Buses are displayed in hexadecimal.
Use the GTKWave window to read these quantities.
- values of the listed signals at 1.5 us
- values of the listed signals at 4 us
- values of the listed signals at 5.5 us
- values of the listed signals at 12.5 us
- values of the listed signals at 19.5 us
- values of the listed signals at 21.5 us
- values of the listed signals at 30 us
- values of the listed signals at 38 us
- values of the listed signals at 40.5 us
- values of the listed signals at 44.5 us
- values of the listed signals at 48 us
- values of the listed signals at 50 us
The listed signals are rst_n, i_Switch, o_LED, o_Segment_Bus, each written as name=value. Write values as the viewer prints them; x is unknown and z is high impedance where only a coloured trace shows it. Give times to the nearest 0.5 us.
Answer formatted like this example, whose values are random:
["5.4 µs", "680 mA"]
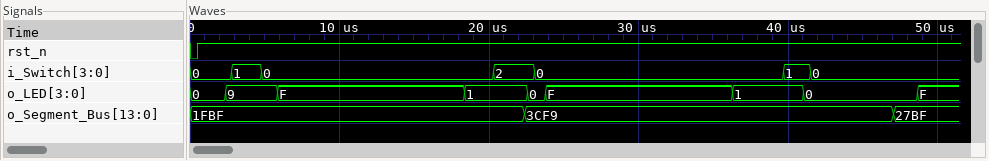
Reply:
["rst_n=1, i_Switch=0, o_LED=0, o_Segment_Bus=1FBF", "rst_n=1, i_Switch=1, o_LED=9, o_Segment_Bus=1FBF", "rst_n=1, i_Switch=0, o_LED=9, o_Segment_Bus=1FBF", "rst_n=1, i_Switch=0, o_LED=F, o_Segment_Bus=1FBF", "rst_n=1, i_Switch=0, o_LED=1, o_Segment_Bus=1FBF", "rst_n=1, i_Switch=2, o_LED=1, o_Segment_Bus=1FBF", "rst_n=1, i_Switch=0, o_LED=F, o_Segment_Bus=3CF9", "rst_n=1, i_Switch=0, o_LED=1, o_Segment_Bus=3CF9", "rst_n=1, i_Switch=1, o_LED=1, o_Segment_Bus=3CF9", "rst_n=1, i_Switch=0, o_LED=0, o_Segment_Bus=3CF9", "rst_n=1, i_Switch=0, o_LED=0, o_Segment_Bus=27BF", "rst_n=1, i_Switch=0, o_LED=F, o_Segment_Bus=27BF"]
